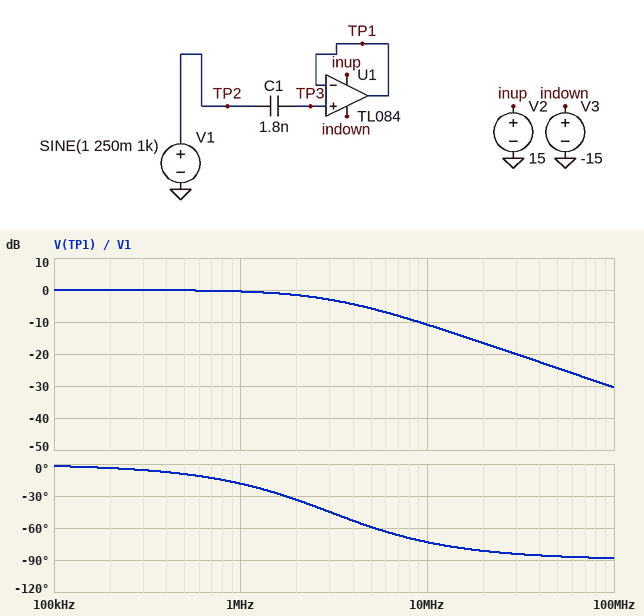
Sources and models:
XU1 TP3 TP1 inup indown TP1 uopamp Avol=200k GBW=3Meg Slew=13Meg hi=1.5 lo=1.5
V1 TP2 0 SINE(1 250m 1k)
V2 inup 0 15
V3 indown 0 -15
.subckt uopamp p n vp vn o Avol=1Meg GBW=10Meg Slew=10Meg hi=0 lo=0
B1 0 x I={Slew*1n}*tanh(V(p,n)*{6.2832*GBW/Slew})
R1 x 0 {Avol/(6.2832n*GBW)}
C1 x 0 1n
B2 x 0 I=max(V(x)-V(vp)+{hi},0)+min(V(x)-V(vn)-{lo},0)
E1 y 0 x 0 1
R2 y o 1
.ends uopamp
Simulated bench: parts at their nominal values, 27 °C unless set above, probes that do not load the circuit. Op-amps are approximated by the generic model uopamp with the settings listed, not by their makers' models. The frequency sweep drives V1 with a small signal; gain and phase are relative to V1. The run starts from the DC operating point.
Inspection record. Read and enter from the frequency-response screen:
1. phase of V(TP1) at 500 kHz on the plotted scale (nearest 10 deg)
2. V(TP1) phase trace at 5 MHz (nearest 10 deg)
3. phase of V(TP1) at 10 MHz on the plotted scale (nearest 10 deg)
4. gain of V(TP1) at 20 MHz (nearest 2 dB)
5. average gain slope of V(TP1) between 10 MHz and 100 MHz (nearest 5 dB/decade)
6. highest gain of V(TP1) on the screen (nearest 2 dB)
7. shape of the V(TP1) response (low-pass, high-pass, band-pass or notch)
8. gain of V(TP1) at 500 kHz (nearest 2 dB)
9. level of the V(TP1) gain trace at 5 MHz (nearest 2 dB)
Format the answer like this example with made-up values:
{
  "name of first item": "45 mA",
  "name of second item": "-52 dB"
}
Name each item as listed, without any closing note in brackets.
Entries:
{
  "phase of V(TP1) at 500 kHz on the plotted scale": "-10 deg",
  "V(TP1) phase trace at 5 MHz": "-60 deg",
  "phase of V(TP1) at 10 MHz on the plotted scale": "-70 deg",
  "gain of V(TP1) at 20 MHz": "-16 dB",
  "average gain slope of V(TP1) between 10 MHz and 100 MHz": "-20 dB/decade",
  "highest gain of V(TP1) on the screen": "0 dB",
  "shape of the V(TP1) response": "low-pass",
  "gain of V(TP1) at 500 kHz": "0 dB",
  "level of the V(TP1) gain trace at 5 MHz": "-6 dB"
}
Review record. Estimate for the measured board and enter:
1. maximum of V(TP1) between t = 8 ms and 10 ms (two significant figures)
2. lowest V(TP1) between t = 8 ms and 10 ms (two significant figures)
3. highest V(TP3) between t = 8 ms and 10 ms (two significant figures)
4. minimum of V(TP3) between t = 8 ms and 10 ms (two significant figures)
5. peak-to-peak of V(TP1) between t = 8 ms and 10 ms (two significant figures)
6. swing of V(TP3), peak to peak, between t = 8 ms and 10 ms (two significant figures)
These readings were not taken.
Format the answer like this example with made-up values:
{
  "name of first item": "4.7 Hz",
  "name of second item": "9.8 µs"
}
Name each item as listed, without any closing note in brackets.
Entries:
{
  "maximum of V(TP1) between t = 8 ms and 10 ms": "250 mV",
  "lowest V(TP1) between t = 8 ms and 10 ms": "-250 mV",
  "highest V(TP3) between t = 8 ms and 10 ms": "250 mV",
  "minimum of V(TP3) between t = 8 ms and 10 ms": "-250 mV",
  "peak-to-peak of V(TP1) between t = 8 ms and 10 ms": "500 mV",
  "swing of V(TP3), peak to peak, between t = 8 ms and 10 ms": "500 mV"
}
